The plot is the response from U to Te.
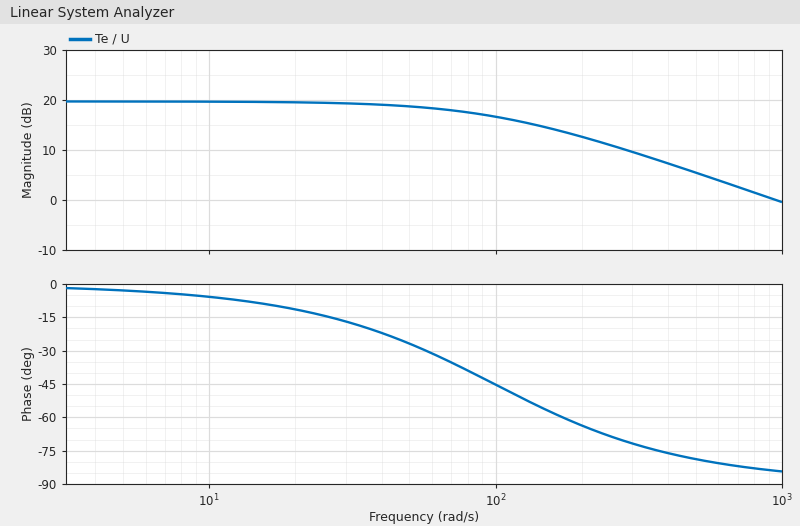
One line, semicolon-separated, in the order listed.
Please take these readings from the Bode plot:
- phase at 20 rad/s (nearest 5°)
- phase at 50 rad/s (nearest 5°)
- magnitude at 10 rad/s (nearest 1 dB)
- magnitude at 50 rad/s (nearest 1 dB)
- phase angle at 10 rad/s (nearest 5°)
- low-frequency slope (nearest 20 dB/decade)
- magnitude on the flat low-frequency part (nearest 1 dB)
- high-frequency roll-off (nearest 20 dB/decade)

-10°; -25°; 20 dB; 19 dB; -5°; 0 dB/decade; 20 dB; -20 dB/decade
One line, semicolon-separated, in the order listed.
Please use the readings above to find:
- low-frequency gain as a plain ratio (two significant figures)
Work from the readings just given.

10
